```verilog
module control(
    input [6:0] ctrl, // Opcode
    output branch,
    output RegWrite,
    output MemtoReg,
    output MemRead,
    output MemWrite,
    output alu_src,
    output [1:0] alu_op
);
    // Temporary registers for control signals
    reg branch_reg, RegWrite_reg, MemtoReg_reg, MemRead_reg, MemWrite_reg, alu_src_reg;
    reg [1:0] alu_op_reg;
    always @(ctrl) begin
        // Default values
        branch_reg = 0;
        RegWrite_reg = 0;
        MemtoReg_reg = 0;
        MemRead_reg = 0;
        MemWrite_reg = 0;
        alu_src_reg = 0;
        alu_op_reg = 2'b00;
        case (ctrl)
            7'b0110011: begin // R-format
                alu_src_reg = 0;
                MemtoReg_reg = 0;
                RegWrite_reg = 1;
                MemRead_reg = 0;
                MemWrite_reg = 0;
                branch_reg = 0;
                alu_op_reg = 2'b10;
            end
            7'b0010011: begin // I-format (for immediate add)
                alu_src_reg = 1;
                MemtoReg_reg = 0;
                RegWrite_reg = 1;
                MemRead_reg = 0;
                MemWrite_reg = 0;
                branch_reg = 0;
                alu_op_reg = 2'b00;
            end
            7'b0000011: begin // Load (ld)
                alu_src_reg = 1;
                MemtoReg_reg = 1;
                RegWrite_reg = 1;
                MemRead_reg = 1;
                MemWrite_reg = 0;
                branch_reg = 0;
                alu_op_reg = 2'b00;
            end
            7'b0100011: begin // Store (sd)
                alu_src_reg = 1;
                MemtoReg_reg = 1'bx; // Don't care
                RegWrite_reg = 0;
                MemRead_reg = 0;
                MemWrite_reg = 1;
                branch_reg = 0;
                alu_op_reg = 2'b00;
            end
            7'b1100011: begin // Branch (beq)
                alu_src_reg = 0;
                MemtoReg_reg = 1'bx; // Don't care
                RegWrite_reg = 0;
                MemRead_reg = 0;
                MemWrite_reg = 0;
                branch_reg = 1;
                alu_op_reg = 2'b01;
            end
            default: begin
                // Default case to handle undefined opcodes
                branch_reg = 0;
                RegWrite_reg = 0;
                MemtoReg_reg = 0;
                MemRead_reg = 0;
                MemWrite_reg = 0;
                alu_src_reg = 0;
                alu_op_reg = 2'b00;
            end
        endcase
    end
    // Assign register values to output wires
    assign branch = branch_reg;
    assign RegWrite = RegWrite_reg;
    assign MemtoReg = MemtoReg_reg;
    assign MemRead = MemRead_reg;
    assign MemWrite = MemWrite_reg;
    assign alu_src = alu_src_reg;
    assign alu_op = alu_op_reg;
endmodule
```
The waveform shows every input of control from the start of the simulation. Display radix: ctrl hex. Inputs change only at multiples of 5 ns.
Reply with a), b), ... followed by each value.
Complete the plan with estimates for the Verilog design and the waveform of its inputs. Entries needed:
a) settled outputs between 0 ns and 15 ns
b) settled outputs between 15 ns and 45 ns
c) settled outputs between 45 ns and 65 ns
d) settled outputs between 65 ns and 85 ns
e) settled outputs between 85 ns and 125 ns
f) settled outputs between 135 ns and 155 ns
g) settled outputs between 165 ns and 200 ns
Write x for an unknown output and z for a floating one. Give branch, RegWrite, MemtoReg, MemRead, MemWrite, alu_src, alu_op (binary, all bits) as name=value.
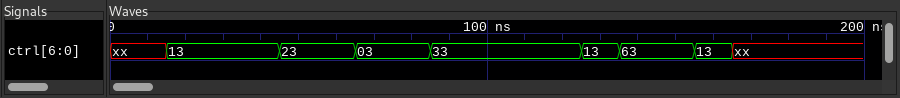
a) branch=x, RegWrite=x, MemtoReg=x, MemRead=x, MemWrite=x, alu_src=x, alu_op=x
b) branch=0, RegWrite=1, MemtoReg=0, MemRead=0, MemWrite=0, alu_src=1, alu_op=00
c) branch=0, RegWrite=0, MemtoReg=x, MemRead=0, MemWrite=1, alu_src=1, alu_op=00
d) branch=0, RegWrite=1, MemtoReg=1, MemRead=1, MemWrite=0, alu_src=1, alu_op=00
e) branch=0, RegWrite=1, MemtoReg=0, MemRead=0, MemWrite=0, alu_src=0, alu_op=10
f) branch=1, RegWrite=0, MemtoReg=x, MemRead=0, MemWrite=0, alu_src=0, alu_op=01
g) branch=0, RegWrite=0, MemtoReg=0, MemRead=0, MemWrite=0, alu_src=0, alu_op=00
